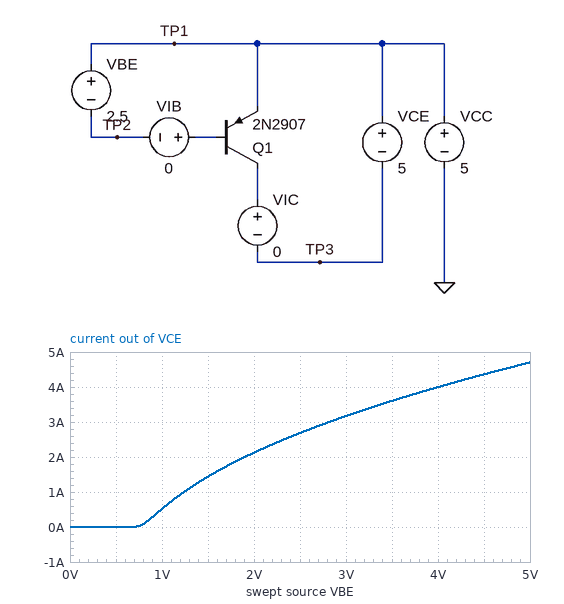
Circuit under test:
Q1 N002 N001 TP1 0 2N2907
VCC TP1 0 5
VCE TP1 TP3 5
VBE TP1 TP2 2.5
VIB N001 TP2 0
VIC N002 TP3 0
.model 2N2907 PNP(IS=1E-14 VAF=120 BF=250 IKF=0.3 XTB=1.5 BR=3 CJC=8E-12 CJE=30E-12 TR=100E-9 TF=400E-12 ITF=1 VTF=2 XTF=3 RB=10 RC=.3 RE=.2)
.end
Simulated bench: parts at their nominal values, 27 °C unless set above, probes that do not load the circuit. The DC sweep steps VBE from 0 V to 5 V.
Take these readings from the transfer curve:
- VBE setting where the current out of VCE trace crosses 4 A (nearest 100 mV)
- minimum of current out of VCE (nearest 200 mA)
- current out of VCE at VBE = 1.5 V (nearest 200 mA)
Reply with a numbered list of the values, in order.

1. 4.0 V
2. 0 A
3. 1.4 A
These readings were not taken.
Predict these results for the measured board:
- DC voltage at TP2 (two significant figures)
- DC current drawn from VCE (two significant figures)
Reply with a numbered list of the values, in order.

1. 2.5 V
2. 2.7 A
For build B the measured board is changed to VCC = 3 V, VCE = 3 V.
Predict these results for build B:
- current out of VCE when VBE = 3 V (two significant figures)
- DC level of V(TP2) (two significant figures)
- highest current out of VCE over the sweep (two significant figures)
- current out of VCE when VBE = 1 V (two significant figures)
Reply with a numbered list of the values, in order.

1. 3.1 A
2. 500 mV
3. 4.6 A
4. 510 mA
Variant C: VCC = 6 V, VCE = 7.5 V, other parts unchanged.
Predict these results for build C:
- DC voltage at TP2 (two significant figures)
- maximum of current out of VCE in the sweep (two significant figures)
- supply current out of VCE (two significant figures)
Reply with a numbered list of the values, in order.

1. 3.5 V
2. 4.8 A
3. 2.7 A
